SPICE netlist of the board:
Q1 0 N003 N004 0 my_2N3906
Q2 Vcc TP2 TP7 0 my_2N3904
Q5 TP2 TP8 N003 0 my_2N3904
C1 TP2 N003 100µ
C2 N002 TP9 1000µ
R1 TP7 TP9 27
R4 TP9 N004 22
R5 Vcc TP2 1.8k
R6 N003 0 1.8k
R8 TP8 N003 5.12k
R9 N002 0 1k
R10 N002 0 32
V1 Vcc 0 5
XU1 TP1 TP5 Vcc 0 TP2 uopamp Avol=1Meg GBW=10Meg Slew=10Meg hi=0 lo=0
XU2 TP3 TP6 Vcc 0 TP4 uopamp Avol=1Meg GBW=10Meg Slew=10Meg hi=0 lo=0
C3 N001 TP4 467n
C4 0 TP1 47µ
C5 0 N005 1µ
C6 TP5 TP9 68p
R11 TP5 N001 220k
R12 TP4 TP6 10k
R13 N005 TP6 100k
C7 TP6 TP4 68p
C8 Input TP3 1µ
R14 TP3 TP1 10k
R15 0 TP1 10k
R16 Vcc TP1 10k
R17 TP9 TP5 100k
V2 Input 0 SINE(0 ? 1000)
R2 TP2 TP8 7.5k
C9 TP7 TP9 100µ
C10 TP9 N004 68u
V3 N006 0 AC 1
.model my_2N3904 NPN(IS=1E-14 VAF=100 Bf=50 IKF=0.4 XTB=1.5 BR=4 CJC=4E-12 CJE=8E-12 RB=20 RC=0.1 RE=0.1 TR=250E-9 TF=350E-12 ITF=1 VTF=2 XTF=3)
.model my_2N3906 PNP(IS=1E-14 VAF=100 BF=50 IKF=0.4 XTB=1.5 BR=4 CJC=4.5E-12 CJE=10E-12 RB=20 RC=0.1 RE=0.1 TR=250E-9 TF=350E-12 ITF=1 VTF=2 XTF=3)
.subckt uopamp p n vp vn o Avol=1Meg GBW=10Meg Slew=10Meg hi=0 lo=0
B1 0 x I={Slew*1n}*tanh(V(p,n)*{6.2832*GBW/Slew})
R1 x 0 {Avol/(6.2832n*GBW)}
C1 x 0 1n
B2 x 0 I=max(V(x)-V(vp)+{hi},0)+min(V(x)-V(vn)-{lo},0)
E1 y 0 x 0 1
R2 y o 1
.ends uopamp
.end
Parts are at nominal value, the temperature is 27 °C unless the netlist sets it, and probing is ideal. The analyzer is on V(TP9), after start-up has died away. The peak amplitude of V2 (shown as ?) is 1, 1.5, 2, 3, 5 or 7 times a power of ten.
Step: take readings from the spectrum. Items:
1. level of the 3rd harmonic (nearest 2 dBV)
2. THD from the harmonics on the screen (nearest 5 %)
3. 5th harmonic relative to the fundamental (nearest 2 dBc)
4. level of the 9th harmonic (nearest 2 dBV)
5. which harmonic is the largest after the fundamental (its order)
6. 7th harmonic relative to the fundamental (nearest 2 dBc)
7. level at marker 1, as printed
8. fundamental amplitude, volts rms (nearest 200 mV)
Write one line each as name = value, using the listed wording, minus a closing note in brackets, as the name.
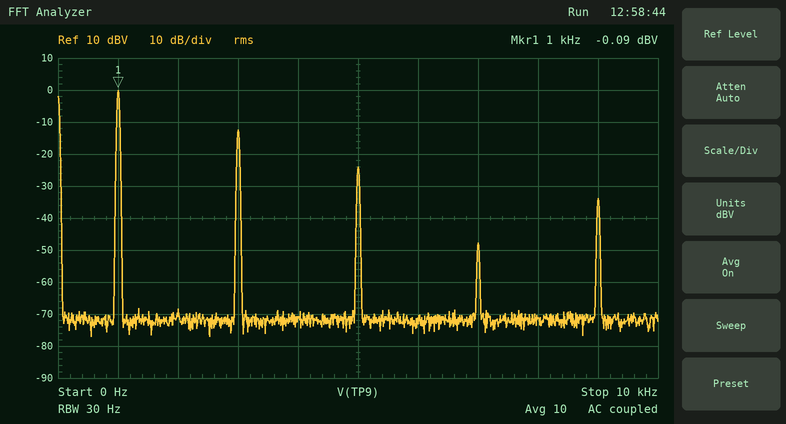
level of the 3rd harmonic = -12 dBV
THD from the harmonics on the screen = 25 %
5th harmonic relative to the fundamental = -24 dBc
level of the 9th harmonic = -34 dBV
which harmonic is the largest after the fundamental = 3
7th harmonic relative to the fundamental = -48 dBc
level at marker 1, as printed = -0.09 dBV
fundamental amplitude, volts rms = 1.0 V
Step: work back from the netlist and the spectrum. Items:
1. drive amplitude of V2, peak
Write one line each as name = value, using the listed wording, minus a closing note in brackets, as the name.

drive amplitude of V2, peak = 5 V
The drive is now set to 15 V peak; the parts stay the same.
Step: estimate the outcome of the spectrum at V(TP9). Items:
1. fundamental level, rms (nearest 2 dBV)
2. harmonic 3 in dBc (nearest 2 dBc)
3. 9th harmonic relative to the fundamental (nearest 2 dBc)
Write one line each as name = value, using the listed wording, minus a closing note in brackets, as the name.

fundamental level, rms = 0 dBV
harmonic 3 in dBc = -10 dBc
9th harmonic relative to the fundamental = -22 dBc
